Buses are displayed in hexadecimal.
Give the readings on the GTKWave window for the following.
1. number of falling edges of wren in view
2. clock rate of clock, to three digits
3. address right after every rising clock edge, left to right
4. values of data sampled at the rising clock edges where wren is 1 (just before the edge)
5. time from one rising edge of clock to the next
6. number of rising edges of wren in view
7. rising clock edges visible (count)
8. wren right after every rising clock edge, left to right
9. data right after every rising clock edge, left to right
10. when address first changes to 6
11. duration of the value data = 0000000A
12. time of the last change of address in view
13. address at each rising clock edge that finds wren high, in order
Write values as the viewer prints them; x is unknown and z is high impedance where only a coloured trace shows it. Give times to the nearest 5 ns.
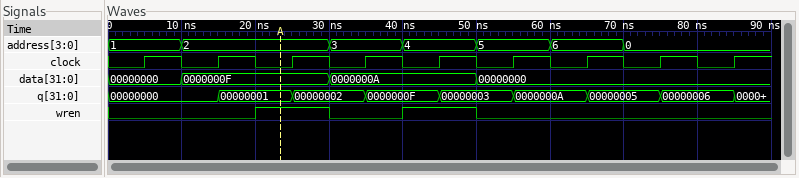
2
100 MHz
1, 2, 2, 3, 4, 5, 6, 0, 0
0000000F, 0000000A
10 ns
2
9
0 0 1 0 1 0 0 0 0
00000000, 0000000F, 0000000F, 0000000A, 0000000A, 00000000, 00000000, 00000000, 00000000
60 ns
20 ns
70 ns
2, 4
